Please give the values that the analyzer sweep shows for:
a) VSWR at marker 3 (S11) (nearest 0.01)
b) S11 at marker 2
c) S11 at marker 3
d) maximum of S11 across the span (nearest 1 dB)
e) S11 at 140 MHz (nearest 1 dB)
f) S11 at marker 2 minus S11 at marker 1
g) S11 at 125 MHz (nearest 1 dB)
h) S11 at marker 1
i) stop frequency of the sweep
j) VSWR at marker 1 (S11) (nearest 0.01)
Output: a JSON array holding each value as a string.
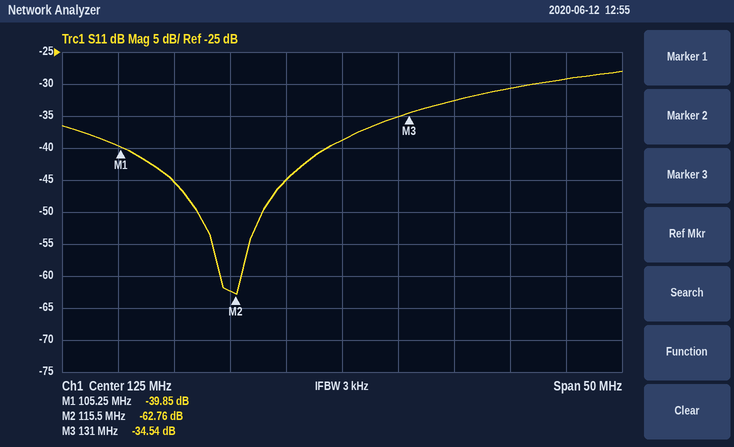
["1.04", "-62.76 dB", "-34.54 dB", "-28 dB", "-31 dB", "-22.91 dB", "-39 dB", "-39.85 dB", "150 MHz", "1.02"]
